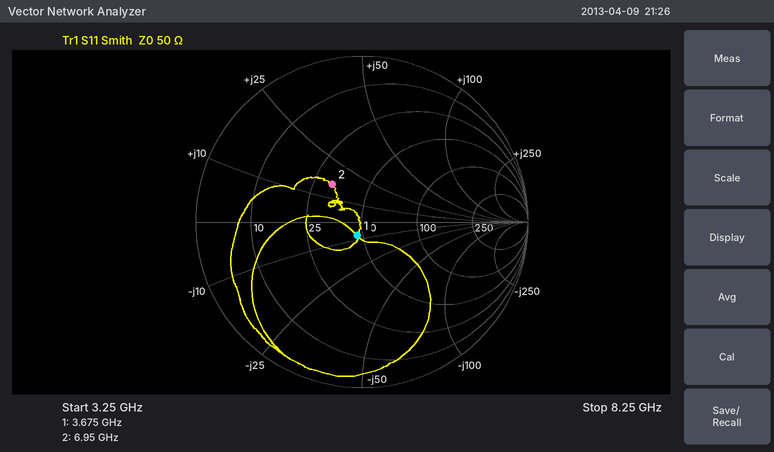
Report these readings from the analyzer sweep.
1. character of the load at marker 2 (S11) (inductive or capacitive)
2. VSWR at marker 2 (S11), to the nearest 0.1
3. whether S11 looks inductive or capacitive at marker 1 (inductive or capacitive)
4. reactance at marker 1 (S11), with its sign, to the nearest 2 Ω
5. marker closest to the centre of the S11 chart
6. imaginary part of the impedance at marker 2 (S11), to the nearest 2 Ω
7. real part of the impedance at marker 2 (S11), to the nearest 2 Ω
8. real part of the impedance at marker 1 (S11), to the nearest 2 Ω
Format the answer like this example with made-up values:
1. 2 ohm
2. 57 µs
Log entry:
1. inductive
2. 1.8
3. capacitive
4. -8 Ω
5. marker 1
6. +16 Ω
7. 32 Ω
8. 46 Ω
